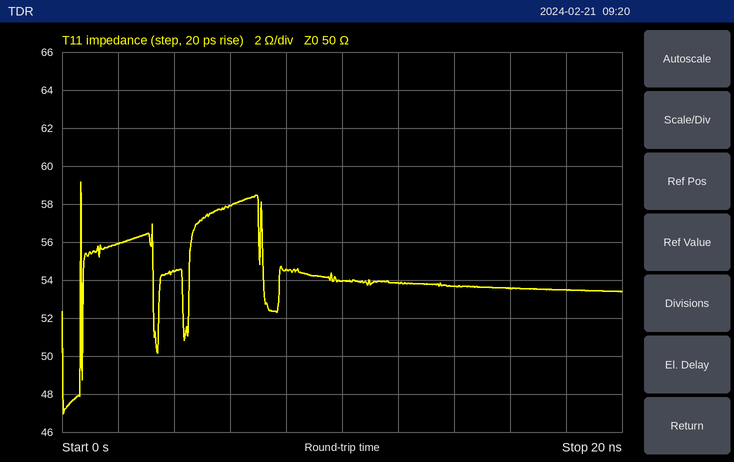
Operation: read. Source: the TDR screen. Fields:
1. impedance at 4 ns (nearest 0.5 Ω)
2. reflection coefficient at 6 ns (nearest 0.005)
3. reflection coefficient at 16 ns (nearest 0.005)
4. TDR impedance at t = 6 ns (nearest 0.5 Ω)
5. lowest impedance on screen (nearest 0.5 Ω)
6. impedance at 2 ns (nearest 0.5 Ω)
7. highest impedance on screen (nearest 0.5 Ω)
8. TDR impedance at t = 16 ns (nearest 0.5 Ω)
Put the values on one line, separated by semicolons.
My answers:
54.5 Ω; +0.075; +0.035; 58.0 Ω; 47.0 Ω; 56.0 Ω; 59.0 Ω; 53.5 Ω
